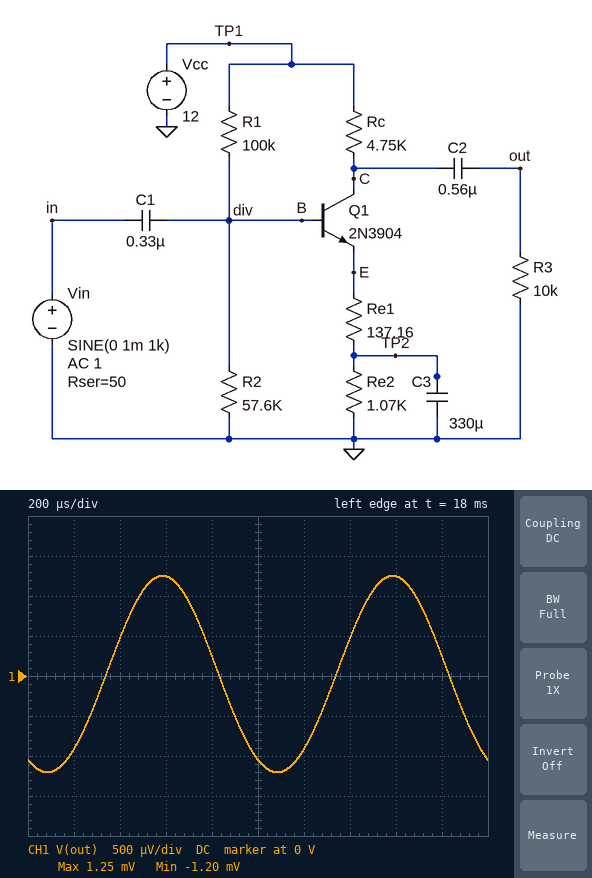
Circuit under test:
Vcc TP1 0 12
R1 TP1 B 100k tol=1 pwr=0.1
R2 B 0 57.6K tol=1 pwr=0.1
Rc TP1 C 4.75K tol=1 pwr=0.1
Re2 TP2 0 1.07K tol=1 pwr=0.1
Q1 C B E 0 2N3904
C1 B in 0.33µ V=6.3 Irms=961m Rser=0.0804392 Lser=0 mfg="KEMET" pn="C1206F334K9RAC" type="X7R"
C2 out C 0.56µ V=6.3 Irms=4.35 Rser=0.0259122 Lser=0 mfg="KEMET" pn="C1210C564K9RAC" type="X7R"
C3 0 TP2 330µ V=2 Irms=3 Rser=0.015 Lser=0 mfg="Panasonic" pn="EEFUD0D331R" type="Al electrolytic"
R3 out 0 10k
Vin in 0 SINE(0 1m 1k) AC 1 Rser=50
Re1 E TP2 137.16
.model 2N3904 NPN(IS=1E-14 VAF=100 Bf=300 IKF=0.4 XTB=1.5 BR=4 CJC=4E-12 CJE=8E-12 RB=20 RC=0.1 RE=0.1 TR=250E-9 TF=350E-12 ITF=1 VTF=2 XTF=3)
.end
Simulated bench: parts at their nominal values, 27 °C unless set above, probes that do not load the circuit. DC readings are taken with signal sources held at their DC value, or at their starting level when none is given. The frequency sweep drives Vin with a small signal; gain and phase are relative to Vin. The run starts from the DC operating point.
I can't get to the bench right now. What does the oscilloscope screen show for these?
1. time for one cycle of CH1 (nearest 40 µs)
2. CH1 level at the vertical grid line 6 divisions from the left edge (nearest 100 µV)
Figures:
1.00 ms
-900 µV
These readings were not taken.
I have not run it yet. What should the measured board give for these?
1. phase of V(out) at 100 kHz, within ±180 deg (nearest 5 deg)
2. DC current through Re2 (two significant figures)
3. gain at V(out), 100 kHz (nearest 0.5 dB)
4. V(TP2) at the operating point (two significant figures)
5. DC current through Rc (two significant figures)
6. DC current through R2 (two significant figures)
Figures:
150 deg
2.0 mA
6.5 dB
2.2 V
2.0 mA
54 µA
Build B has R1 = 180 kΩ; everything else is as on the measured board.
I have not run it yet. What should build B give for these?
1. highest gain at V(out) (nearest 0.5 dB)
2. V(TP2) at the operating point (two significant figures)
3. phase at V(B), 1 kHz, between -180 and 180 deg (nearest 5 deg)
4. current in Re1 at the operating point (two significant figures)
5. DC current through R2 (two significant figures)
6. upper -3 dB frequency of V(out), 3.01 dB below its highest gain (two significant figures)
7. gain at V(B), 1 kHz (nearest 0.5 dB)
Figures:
26.5 dB
1.8 V
0 deg
1.7 mA
46 µA
12 MHz
0 dB
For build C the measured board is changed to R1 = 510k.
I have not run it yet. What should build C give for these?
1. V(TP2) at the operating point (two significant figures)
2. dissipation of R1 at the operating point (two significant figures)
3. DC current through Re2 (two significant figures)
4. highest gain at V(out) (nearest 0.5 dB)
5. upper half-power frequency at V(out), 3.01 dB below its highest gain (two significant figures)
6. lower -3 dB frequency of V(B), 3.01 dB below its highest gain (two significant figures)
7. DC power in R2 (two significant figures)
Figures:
460 mV
230 µW
430 µA
24.0 dB
20 MHz
18 Hz
23 µW
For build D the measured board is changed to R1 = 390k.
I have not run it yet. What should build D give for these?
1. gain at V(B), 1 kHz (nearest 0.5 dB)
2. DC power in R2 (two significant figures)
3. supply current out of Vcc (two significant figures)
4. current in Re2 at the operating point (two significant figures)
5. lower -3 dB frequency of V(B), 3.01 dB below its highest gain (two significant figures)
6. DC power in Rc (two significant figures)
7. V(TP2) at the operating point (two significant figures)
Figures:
0 dB
36 µW
690 µA
660 µA
19 Hz
2.1 mW
710 mV
